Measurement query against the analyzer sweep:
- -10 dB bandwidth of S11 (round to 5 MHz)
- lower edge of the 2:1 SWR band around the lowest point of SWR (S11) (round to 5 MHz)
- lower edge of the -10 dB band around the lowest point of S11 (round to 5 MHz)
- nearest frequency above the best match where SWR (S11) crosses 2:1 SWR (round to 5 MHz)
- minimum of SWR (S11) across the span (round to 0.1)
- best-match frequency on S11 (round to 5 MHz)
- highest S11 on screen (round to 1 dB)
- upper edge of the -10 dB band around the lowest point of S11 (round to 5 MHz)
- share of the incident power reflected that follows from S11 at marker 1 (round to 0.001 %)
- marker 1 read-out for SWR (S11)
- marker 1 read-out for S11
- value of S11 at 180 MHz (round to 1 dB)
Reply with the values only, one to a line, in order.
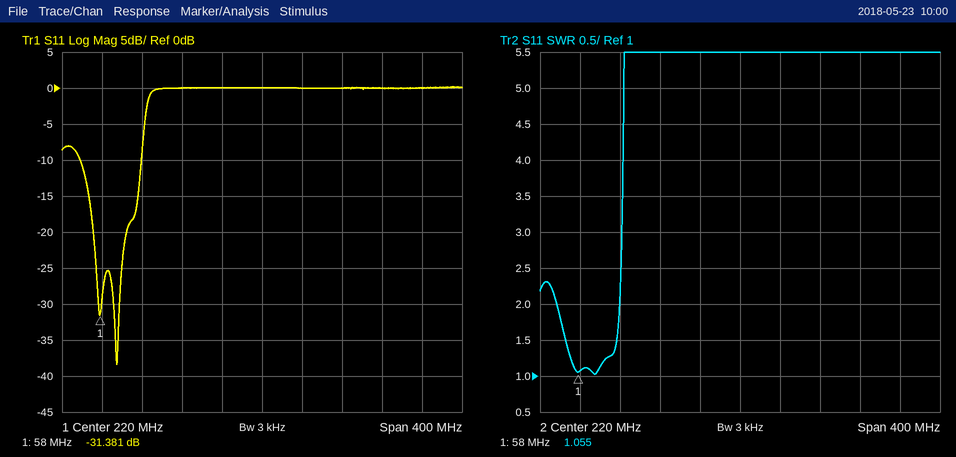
60 MHz
35 MHz
40 MHz
100 MHz
1.0
75 MHz
0 dB
100 MHz
0.073 %
1.055
-31.381 dB
0 dB
